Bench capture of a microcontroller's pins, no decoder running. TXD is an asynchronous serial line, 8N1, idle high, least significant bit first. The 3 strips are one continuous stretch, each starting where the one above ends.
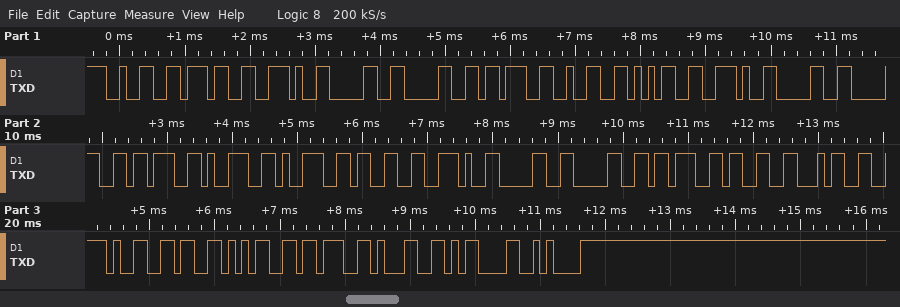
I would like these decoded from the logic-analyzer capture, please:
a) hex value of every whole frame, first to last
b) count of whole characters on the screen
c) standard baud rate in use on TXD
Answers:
32 37 2E 30 30 3B 32 35 2E 30 30 3B 39 39 33 2E 30 30 3B 33 34 2E 36 35 3B 31 0D 0A
28
9600 baud
